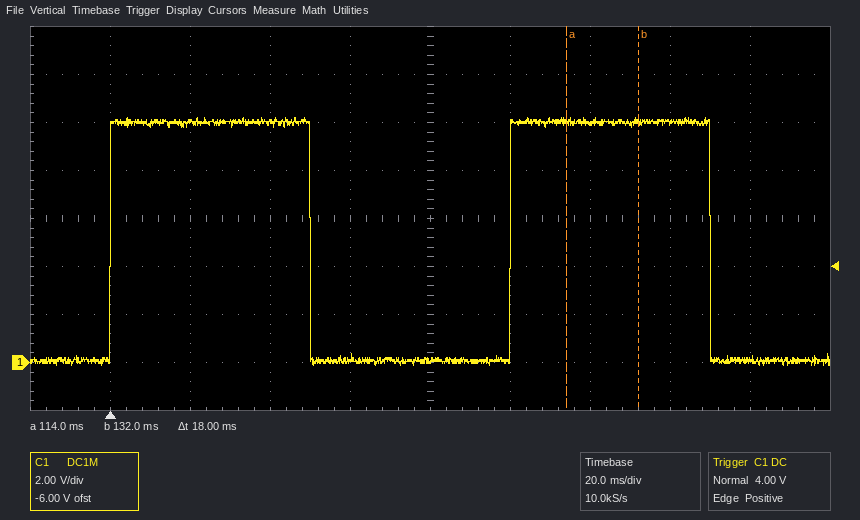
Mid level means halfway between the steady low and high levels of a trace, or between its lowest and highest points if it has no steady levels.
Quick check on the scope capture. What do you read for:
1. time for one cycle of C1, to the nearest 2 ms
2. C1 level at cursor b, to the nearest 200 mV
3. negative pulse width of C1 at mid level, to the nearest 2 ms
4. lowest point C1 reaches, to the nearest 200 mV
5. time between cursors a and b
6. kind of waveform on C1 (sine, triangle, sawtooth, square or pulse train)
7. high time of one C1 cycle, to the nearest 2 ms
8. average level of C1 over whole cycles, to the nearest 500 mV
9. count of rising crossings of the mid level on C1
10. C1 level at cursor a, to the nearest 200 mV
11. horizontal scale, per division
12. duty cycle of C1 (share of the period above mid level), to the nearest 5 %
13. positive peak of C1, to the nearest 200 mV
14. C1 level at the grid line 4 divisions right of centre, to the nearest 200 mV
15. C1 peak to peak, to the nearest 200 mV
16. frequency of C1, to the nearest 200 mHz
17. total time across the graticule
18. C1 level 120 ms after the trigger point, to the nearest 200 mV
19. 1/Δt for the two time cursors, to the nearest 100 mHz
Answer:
100 ms
10.0 V
50 ms
-200 mV
18 ms
square
50 ms
5.0 V
2
10.0 V
20 ms
50 %
10.2 V
200 mV
10.4 V
10.0 Hz
200 ms
10.0 V
55.6 Hz
